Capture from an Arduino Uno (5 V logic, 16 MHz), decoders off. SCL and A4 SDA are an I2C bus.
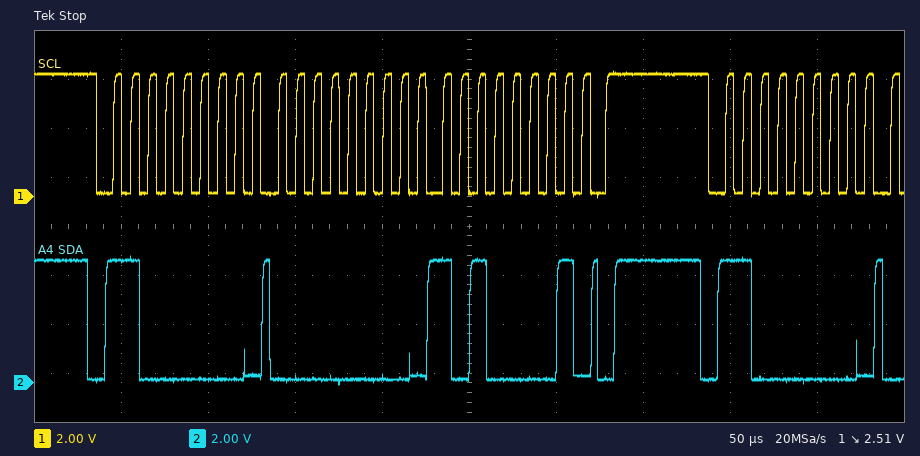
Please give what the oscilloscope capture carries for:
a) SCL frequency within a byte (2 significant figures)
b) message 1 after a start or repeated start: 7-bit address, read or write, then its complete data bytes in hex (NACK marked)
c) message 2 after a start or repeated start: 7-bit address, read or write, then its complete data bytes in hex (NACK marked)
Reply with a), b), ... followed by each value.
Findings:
a) 100 kHz
b) 0x60 write: 00 A1
c) 0x60 write
